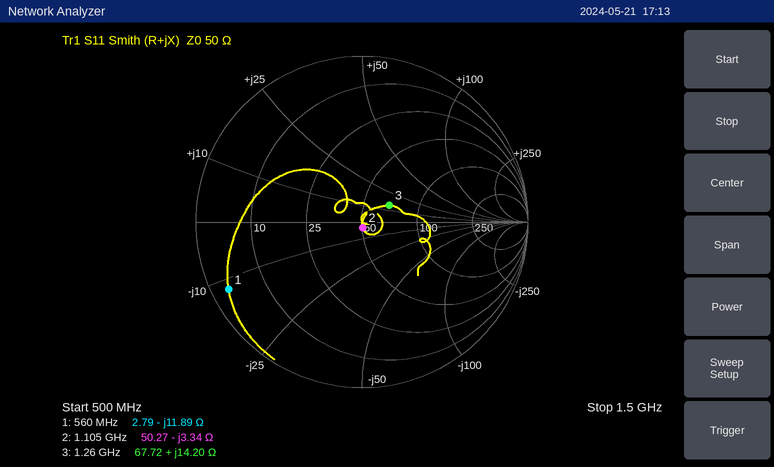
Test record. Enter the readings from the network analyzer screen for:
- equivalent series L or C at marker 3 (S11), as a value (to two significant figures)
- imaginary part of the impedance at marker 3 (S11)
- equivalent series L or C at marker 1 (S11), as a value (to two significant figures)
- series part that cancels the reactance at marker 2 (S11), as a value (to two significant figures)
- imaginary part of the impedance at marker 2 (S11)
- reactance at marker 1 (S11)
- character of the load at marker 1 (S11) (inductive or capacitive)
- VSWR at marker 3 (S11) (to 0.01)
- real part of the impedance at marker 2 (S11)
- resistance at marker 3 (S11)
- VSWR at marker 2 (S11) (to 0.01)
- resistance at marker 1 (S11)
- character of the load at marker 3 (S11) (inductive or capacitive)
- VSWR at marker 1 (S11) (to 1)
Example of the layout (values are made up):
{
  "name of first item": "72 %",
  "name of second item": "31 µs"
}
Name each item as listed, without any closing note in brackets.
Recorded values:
{
  "equivalent series L or C at marker 3 (S11), as a value": "1.8 nH",
  "imaginary part of the impedance at marker 3": "+14.20 Ω",
  "equivalent series L or C at marker 1 (S11), as a value": "24 pF",
  "series part that cancels the reactance at marker 2 (S11), as a value": "480 pH",
  "imaginary part of the impedance at marker 2": "-3.34 Ω",
  "reactance at marker 1": "-11.89 Ω",
  "character of the load at marker 1 (S11)": "capacitive",
  "VSWR at marker 3 (S11)": "1.47",
  "real part of the impedance at marker 2": "50.27 Ω",
  "resistance at marker 3": "67.72 Ω",
  "VSWR at marker 2 (S11)": "1.07",
  "resistance at marker 1": "2.79 Ω",
  "character of the load at marker 3 (S11)": "inductive",
  "VSWR at marker 1 (S11)": "19"
}
